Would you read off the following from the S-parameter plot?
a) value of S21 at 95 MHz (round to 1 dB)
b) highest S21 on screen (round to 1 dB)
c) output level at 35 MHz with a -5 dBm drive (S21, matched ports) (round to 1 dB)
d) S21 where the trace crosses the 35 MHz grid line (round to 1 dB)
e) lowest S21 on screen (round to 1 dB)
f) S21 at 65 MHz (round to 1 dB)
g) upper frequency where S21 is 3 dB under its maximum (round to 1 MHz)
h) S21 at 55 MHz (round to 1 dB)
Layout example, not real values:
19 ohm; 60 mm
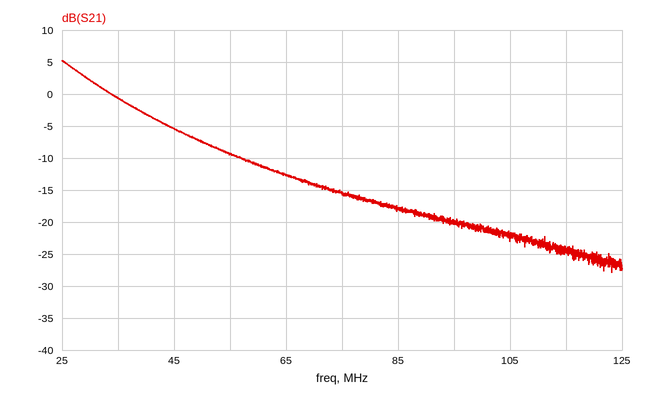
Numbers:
-20 dB; 5 dB; -6 dBm; -1 dB; -28 dB; -13 dB; 30 MHz; -9 dB
